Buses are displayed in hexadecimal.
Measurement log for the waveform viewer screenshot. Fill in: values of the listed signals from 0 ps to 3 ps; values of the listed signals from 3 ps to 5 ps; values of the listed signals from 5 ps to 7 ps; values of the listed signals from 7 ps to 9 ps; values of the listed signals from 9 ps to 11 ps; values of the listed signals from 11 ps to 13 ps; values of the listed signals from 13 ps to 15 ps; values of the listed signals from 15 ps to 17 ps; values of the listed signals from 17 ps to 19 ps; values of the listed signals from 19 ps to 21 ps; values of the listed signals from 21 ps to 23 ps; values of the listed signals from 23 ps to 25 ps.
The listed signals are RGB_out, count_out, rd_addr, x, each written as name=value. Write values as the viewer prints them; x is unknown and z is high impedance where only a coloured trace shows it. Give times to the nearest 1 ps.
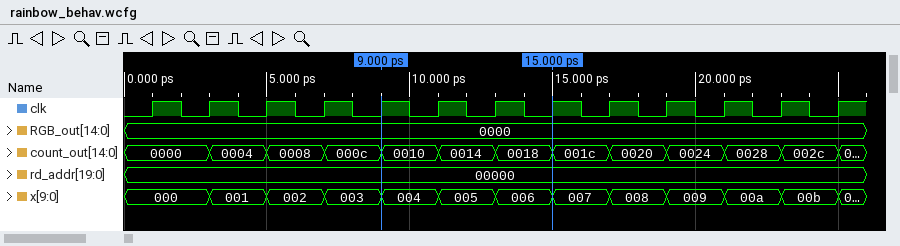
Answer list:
RGB_out=0000, count_out=0000, rd_addr=00000, x=000
RGB_out=0000, count_out=0004, rd_addr=00000, x=001
RGB_out=0000, count_out=0008, rd_addr=00000, x=002
RGB_out=0000, count_out=000c, rd_addr=00000, x=003
RGB_out=0000, count_out=0010, rd_addr=00000, x=004
RGB_out=0000, count_out=0014, rd_addr=00000, x=005
RGB_out=0000, count_out=0018, rd_addr=00000, x=006
RGB_out=0000, count_out=001c, rd_addr=00000, x=007
RGB_out=0000, count_out=0020, rd_addr=00000, x=008
RGB_out=0000, count_out=0024, rd_addr=00000, x=009
RGB_out=0000, count_out=0028, rd_addr=00000, x=00a
RGB_out=0000, count_out=002c, rd_addr=00000, x=00b
